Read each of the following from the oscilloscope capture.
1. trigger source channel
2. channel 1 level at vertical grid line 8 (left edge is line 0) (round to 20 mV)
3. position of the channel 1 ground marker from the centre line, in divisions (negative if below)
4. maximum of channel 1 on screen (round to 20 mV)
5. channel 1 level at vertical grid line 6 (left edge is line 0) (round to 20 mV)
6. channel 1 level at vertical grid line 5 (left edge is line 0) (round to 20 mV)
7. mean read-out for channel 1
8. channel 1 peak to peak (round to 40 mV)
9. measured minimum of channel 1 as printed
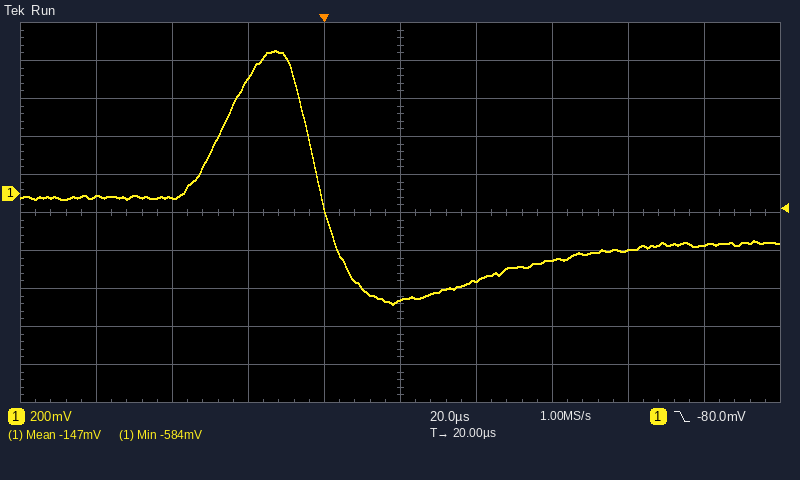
channel 1
-300 mV
+0.5 div
760 mV
-460 mV
-560 mV
-147 mV
1.32 V
-584 mV
